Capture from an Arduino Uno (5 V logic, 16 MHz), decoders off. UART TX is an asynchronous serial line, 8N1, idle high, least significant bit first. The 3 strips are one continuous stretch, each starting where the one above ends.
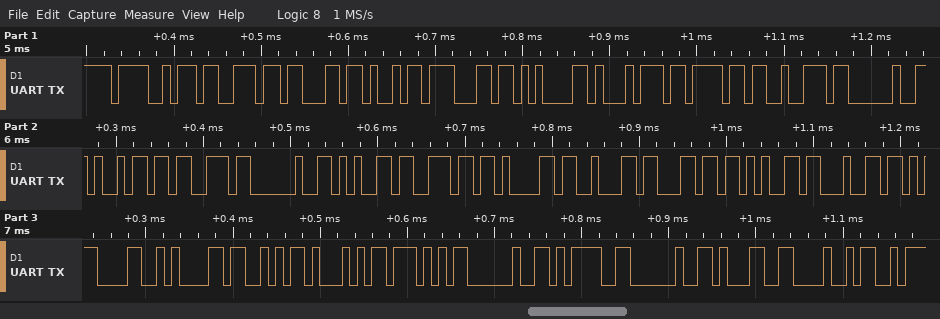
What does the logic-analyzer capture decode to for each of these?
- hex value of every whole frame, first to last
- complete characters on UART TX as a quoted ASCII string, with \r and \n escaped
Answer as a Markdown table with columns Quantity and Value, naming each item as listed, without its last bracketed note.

| Quantity | Value |
|---|---|
| hex value of every whole frame, first to last | 4F 73 63 69 6C 61 74 6F 72 20 69 73 20 65 6E 61 62 6C 65 64 0D 0A 53 51 57 20 3D 20 31 48 |
| complete characters on UART TX as a quoted ASCII string, with \r and \n escaped | "Oscilator is enabled\r\nSQW = 1H" |
